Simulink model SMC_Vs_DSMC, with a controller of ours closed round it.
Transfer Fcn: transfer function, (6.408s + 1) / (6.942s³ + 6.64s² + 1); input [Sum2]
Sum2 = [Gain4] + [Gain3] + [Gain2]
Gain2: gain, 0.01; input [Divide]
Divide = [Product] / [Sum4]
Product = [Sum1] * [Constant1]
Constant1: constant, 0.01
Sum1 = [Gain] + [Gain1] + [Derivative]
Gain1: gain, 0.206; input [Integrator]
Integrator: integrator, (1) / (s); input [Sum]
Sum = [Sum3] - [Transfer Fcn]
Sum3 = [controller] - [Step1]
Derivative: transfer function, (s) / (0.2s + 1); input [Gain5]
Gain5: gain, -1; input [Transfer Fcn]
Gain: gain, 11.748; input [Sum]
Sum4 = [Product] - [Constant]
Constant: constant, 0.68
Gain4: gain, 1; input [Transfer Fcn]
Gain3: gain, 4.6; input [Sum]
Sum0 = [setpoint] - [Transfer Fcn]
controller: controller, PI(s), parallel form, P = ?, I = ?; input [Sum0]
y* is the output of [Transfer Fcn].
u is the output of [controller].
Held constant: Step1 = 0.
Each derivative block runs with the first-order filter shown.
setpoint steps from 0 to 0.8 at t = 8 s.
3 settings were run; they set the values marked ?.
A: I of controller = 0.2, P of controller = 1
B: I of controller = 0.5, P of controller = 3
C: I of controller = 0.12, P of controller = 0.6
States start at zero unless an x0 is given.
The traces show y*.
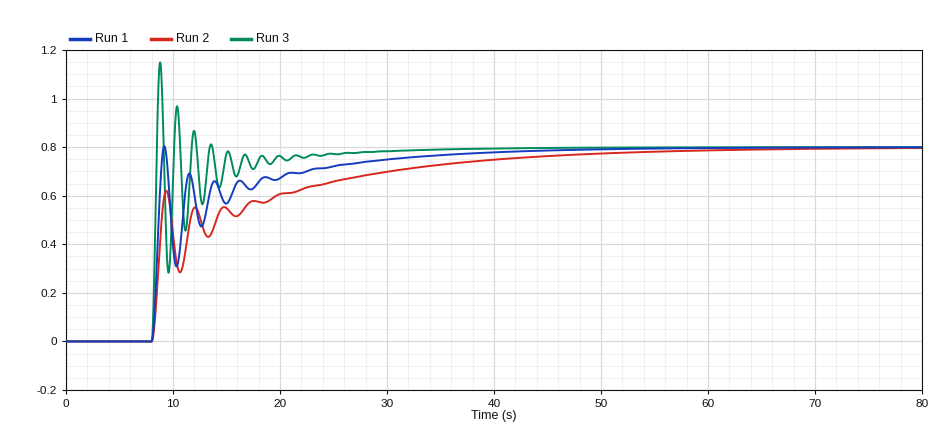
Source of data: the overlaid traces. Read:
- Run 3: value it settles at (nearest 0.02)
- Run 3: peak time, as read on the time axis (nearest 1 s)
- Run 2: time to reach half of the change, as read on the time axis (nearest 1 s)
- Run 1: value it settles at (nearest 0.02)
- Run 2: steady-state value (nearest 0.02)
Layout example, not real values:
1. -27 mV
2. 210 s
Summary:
1. 0.80
2. 9 s
3. 9 s
4. 0.80
5. 0.80
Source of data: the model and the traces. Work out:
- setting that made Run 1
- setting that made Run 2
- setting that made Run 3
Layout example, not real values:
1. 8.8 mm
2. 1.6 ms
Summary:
1. A
2. C
3. B
